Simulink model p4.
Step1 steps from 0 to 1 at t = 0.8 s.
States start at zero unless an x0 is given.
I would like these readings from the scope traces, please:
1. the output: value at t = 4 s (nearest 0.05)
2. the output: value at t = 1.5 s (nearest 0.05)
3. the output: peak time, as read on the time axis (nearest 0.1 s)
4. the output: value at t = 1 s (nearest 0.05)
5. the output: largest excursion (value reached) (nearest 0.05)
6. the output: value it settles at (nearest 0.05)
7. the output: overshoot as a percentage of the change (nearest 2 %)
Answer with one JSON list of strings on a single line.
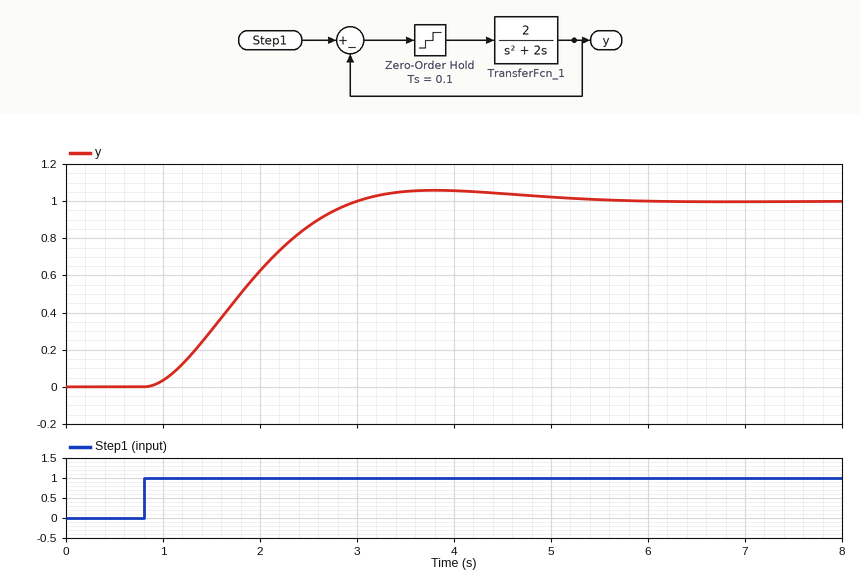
["1.05", "0.30", "3.8 s", "0.05", "1.05", "1.00", "6 %"]
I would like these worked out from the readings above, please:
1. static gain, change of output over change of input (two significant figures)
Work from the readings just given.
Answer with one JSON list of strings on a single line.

["1.0"]
